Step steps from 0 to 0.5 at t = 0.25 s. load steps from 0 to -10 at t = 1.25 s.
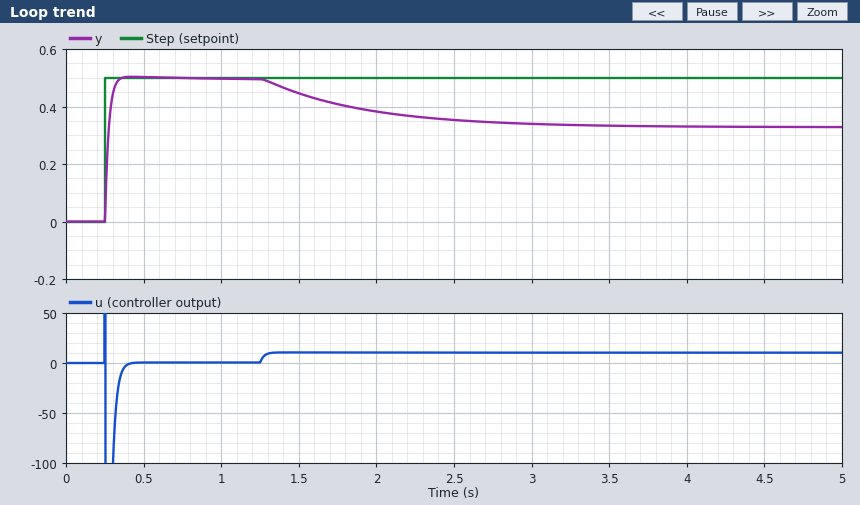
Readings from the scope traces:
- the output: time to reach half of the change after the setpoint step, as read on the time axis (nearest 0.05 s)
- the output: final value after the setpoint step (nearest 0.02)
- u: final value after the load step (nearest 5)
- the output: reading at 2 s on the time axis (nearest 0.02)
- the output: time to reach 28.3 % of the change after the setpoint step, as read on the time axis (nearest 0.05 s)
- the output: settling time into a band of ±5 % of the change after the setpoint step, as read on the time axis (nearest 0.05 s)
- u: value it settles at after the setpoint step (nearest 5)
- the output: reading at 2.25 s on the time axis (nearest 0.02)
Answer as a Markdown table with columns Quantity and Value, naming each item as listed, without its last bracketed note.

| Quantity | Value |
|---|---|
| the output: time to reach half of the change after the setpoint step, as read on the time axis | 0.25 s |
| the output: final value after the setpoint step | 0.50 |
| u: final value after the load step | 10 |
| the output: reading at 2 s on the time axis | 0.38 |
| the output: time to reach 28.3 % of the change after the setpoint step, as read on the time axis | 0.25 s |
| the output: settling time into a band of ±5 % of the change after the setpoint step, as read on the time axis | 0.30 s |
| u: value it settles at after the setpoint step | 0 |
| the output: reading at 2.25 s on the time axis | 0.36 |
